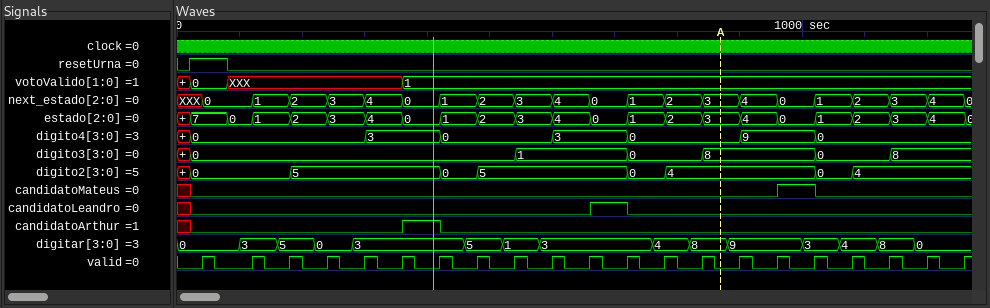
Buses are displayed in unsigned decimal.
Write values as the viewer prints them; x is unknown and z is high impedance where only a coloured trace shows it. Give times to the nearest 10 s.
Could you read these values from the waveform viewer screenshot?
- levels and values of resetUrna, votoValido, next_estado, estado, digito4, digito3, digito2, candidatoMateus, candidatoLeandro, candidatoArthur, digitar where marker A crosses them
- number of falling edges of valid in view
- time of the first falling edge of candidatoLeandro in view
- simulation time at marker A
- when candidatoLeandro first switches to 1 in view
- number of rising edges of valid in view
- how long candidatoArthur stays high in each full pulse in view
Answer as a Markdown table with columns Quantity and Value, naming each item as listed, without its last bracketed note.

| Quantity | Value |
|---|---|
| levels and values of resetUrna, votoValido, next_estado, estado, digito4, digito3, digito2, candidatoMateus, candidatoLeandro, candidatoArthur, digitar where marker A crosses them | resetUrna=0, votoValido=1, next_estado=3, estado=3, digito4=0, digito3=8, digito2=4, candidatoMateus=0, candidatoLeandro=0, candidatoArthur=0, digitar=8 |
| number of falling edges of valid in view | 20 |
| time of the first falling edge of candidatoLeandro in view | 720 s |
| simulation time at marker A | 870 s |
| when candidatoLeandro first switches to 1 in view | 660 s |
| number of rising edges of valid in view | 21 |
| how long candidatoArthur stays high in each full pulse in view | 60 s |
